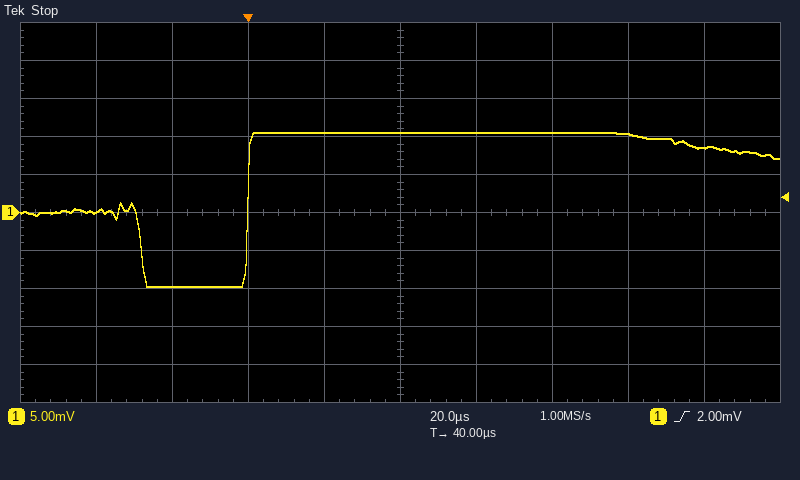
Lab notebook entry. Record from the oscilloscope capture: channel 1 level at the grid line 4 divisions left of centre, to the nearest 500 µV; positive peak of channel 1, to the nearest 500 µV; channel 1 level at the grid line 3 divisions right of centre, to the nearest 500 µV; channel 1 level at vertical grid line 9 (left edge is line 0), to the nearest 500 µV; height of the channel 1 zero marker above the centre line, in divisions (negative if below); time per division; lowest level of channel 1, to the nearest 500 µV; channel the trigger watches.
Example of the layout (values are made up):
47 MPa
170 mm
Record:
0.0 mV
10.5 mV
10.5 mV
8.5 mV
0.0 div
20 µs
-9.5 mV
channel 1
